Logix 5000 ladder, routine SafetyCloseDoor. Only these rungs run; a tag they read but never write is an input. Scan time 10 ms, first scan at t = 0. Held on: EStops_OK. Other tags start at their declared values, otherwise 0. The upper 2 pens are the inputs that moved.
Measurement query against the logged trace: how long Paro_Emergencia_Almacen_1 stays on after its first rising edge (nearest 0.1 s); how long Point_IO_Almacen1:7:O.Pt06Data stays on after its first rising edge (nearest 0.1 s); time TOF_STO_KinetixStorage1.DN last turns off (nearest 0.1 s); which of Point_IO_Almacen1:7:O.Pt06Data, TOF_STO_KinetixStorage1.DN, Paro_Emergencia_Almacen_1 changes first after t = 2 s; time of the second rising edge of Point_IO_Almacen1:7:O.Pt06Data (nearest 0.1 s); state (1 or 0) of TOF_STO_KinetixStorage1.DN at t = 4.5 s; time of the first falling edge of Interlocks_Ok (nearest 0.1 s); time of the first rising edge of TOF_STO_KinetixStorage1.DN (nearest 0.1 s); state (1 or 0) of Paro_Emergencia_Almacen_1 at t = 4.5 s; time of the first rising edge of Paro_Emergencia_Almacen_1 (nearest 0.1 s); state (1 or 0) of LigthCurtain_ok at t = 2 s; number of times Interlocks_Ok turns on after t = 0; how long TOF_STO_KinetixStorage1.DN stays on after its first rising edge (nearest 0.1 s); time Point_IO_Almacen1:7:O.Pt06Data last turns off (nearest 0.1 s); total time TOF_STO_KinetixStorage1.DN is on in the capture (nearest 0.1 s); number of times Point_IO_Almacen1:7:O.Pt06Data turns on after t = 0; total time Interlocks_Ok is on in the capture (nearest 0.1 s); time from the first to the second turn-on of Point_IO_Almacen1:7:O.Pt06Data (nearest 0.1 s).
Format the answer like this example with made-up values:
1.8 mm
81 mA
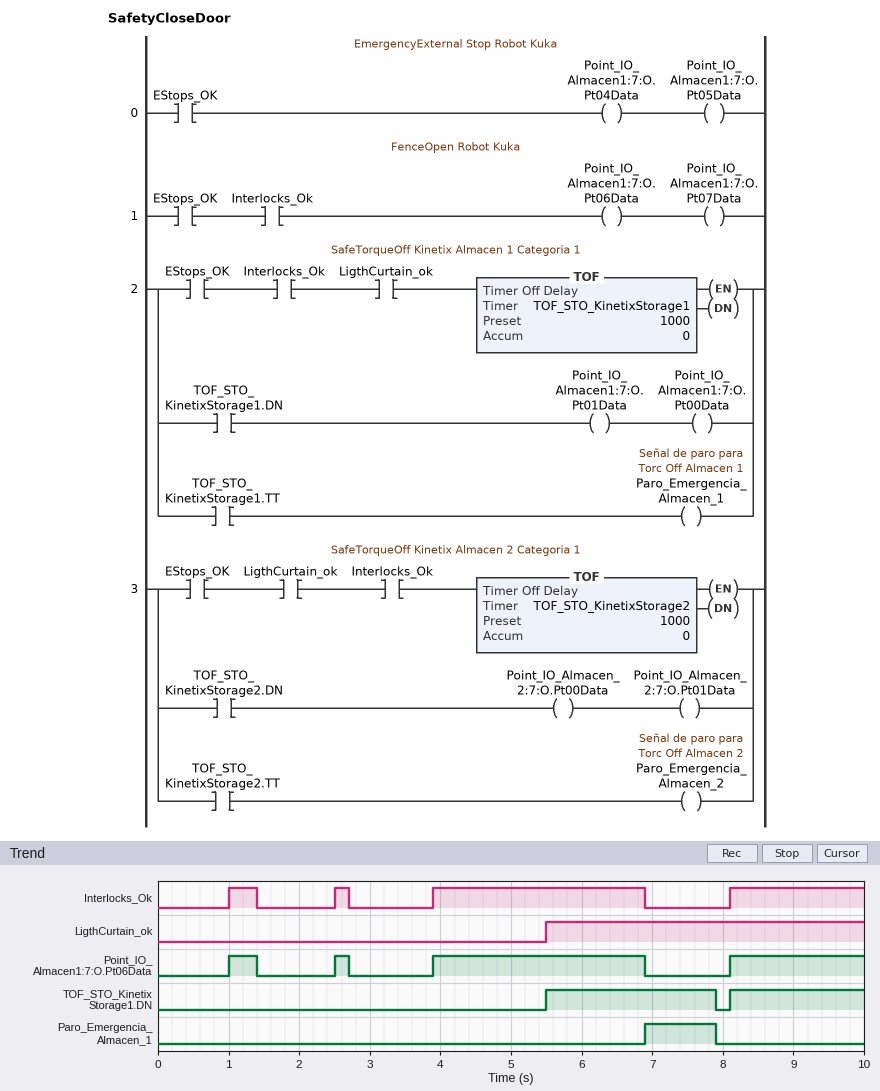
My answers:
1.0 s
0.4 s
7.9 s
Point_IO_Almacen1:7:O.Pt06Data
2.5 s
0
1.4 s
5.5 s
0
6.9 s
0
4
2.4 s
6.9 s
4.3 s
4
5.5 s
1.5 s
